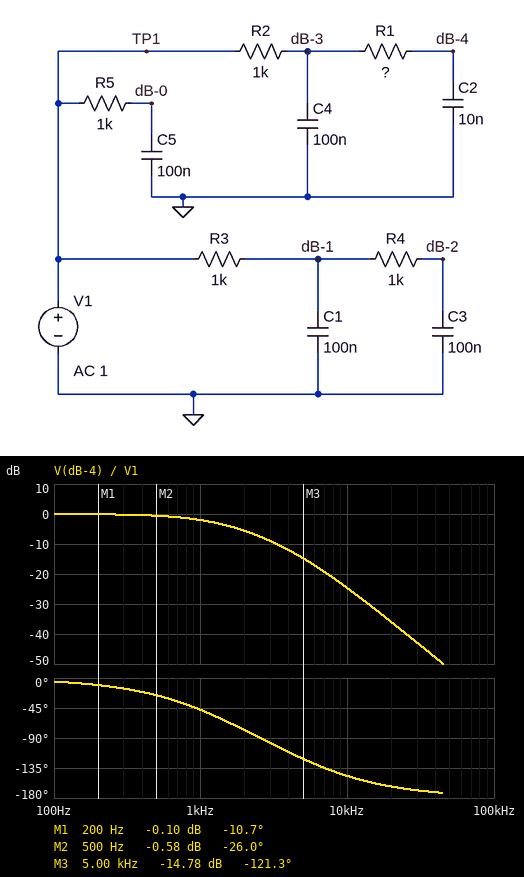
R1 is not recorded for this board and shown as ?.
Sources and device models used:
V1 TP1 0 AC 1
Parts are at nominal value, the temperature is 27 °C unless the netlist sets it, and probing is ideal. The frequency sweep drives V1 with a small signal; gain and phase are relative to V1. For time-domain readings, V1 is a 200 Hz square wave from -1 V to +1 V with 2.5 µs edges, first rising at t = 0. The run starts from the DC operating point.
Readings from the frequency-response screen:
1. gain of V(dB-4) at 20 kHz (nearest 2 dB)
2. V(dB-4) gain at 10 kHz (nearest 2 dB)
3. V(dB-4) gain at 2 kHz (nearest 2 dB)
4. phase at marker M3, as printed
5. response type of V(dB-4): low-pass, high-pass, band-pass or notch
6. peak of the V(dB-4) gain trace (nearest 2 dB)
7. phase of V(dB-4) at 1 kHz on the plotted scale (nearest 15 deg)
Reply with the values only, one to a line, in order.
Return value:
-36 dB
-24 dB
-6 dB
-121.3 deg
low-pass
0 dB
-45 deg
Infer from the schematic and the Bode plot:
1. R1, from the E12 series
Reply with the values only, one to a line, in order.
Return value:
3.9 kΩ
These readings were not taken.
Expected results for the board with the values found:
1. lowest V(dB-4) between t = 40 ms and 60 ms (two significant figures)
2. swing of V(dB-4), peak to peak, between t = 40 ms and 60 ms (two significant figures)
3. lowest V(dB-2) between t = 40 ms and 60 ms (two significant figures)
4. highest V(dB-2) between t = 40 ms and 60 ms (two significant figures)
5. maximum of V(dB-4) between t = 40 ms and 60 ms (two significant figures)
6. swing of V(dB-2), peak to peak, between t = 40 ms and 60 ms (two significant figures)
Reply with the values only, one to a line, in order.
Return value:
-1.0 V
2.0 V
-1.0 V
1.0 V
1.0 V
2.0 V
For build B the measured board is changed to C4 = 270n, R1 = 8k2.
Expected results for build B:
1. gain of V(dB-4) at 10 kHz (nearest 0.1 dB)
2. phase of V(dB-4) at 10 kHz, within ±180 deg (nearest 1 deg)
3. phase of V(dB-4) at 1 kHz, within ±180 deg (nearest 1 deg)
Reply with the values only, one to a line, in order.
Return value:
-39.0 dB
-165 deg
-87 deg
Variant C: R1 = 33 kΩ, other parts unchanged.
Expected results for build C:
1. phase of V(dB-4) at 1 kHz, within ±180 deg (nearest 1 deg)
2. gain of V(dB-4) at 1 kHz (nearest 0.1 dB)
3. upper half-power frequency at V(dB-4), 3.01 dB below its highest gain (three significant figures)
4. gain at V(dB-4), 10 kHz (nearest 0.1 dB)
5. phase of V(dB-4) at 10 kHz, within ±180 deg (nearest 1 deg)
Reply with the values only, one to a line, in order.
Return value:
-96 deg
-8.9 dB
432 Hz
-42.4 dB
-168 deg
